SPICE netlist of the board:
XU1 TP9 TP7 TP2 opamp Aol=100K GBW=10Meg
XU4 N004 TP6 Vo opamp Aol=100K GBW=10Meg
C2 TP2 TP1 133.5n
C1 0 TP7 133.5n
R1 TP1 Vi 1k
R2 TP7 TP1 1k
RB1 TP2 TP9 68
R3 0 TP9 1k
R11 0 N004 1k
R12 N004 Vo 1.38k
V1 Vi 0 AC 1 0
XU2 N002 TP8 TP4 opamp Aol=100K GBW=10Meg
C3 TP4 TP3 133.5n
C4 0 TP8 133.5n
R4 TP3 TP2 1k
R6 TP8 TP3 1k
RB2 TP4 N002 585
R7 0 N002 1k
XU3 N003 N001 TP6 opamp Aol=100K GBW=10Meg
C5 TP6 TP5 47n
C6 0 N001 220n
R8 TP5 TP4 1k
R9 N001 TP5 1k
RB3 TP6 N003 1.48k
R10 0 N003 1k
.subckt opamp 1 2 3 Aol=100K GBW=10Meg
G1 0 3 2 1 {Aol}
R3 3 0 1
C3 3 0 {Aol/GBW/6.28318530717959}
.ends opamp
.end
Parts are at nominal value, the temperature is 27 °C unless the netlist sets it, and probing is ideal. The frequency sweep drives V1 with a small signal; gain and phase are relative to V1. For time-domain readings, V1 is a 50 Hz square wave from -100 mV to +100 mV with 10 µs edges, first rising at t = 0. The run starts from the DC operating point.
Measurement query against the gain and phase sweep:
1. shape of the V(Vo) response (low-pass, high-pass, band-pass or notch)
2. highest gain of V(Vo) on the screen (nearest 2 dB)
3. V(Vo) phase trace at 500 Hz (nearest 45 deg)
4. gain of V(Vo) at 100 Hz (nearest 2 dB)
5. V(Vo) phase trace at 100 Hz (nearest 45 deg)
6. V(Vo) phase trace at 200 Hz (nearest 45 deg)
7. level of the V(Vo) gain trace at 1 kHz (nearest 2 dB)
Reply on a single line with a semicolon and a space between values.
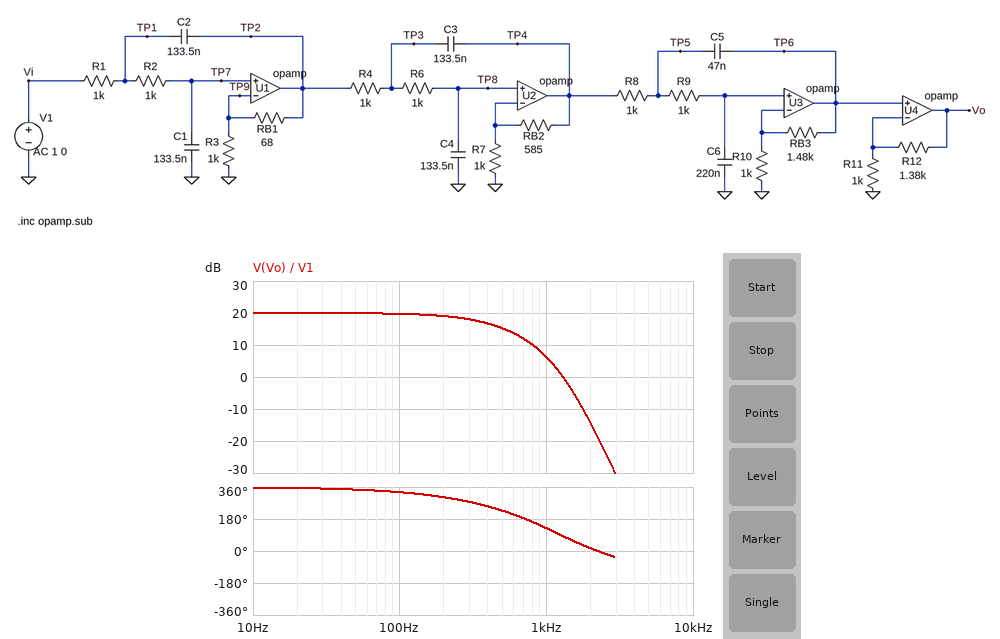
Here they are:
low-pass; 20 dB; 225 deg; 20 dB; 315 deg; 315 deg; 6 dB
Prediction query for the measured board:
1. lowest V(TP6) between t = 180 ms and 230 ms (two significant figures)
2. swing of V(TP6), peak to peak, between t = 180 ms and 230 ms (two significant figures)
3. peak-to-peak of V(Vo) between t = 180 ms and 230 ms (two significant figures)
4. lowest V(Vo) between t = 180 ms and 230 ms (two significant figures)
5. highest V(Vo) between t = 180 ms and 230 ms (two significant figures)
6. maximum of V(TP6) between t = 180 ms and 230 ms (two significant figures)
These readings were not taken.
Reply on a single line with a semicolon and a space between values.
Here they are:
-420 mV; 840 mV; 2.0 V; -1.0 V; 1.0 V; 420 mV
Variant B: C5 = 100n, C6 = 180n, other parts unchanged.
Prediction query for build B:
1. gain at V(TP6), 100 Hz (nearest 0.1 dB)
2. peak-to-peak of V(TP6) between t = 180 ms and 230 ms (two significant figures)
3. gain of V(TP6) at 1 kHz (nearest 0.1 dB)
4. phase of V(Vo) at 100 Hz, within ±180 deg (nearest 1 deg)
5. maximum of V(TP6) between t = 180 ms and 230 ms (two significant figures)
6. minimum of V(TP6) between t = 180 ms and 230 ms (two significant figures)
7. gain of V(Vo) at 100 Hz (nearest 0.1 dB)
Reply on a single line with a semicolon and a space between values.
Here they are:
12.4 dB; 860 mV; 3.7 dB; -24 deg; 430 mV; -430 mV; 19.9 dB
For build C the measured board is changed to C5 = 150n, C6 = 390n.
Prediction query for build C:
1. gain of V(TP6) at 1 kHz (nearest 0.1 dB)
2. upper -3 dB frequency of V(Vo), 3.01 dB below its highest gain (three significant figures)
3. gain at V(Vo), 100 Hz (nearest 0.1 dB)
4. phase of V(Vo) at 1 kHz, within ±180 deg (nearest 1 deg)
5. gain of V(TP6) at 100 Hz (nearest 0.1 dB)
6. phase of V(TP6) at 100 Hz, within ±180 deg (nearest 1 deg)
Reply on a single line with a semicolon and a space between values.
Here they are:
-5.1 dB; 308 Hz; 19.6 dB; 94 deg; 12.1 dB; -36 deg
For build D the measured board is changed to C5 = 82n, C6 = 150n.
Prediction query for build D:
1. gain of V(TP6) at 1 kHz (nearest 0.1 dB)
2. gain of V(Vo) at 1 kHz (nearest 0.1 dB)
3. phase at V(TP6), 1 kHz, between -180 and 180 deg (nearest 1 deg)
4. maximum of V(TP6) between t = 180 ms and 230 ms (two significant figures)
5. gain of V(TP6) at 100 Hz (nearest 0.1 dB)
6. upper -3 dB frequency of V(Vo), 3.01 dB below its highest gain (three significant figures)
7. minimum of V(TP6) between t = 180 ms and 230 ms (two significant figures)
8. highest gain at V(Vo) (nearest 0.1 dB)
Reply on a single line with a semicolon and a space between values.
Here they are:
4.5 dB; 12.1 dB; 139 deg; 430 mV; 12.4 dB; 643 Hz; -430 mV; 20.0 dB
